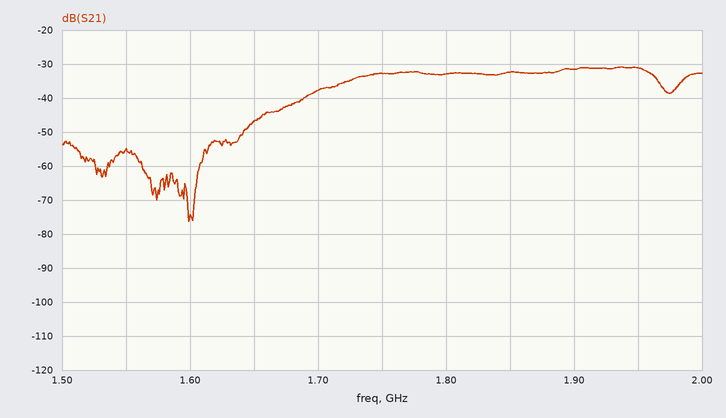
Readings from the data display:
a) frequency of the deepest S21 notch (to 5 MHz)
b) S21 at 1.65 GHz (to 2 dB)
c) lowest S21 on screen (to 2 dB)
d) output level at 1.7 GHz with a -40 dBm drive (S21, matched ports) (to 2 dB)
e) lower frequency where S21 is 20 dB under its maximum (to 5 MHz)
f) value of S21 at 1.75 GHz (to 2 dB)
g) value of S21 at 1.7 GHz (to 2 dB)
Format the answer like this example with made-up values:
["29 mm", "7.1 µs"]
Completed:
["1.600 GHz", "-46 dB", "-76 dB", "-78 dBm", "1.640 GHz", "-32 dB", "-38 dB"]
